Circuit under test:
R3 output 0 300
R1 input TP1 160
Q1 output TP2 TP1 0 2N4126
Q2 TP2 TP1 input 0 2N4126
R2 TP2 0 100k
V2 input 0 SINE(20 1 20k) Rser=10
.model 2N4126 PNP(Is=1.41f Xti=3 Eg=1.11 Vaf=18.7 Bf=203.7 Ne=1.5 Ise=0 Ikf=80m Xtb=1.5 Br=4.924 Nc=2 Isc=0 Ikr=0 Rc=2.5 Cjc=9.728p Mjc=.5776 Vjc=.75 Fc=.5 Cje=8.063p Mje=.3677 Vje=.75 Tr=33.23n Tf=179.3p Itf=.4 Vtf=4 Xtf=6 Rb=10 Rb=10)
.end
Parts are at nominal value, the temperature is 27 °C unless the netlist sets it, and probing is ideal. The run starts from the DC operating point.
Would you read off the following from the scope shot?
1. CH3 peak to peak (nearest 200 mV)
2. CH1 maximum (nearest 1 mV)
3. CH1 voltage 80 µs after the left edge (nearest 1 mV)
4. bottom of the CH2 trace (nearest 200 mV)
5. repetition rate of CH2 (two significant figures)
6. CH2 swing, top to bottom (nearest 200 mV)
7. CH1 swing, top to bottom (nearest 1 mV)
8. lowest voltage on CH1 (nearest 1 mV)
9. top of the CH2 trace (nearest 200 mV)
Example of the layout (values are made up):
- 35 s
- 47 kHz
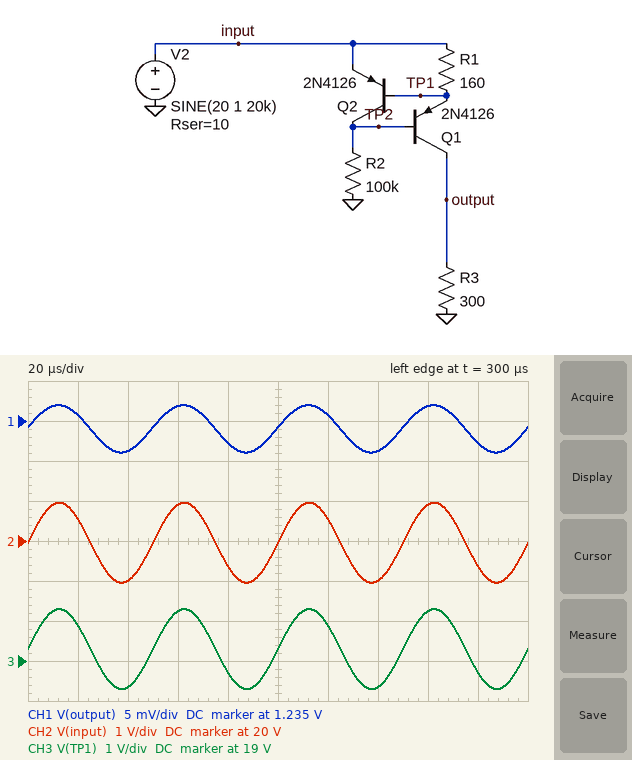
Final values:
- 2.0 V
- 1.237 V
- 1.232 V
- 19.0 V
- 20 kHz
- 2.0 V
- 6 mV
- 1.231 V
- 21.0 V
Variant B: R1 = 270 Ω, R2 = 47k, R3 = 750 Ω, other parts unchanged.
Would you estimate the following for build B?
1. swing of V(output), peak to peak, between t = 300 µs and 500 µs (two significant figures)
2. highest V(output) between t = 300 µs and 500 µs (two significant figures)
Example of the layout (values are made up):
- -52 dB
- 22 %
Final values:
- 8.4 mV
- 1.9 V
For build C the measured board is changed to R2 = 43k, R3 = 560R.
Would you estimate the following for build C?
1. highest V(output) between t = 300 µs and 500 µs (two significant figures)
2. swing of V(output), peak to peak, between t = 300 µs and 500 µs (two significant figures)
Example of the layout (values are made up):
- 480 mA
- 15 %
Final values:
- 2.4 V
- 11 mV
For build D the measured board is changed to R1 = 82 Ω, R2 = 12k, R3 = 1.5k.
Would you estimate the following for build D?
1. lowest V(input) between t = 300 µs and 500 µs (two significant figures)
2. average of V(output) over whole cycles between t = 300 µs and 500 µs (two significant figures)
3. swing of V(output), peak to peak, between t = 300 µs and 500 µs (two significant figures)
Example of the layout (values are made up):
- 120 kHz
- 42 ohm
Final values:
- 19 V
- 13 V
- 60 mV
